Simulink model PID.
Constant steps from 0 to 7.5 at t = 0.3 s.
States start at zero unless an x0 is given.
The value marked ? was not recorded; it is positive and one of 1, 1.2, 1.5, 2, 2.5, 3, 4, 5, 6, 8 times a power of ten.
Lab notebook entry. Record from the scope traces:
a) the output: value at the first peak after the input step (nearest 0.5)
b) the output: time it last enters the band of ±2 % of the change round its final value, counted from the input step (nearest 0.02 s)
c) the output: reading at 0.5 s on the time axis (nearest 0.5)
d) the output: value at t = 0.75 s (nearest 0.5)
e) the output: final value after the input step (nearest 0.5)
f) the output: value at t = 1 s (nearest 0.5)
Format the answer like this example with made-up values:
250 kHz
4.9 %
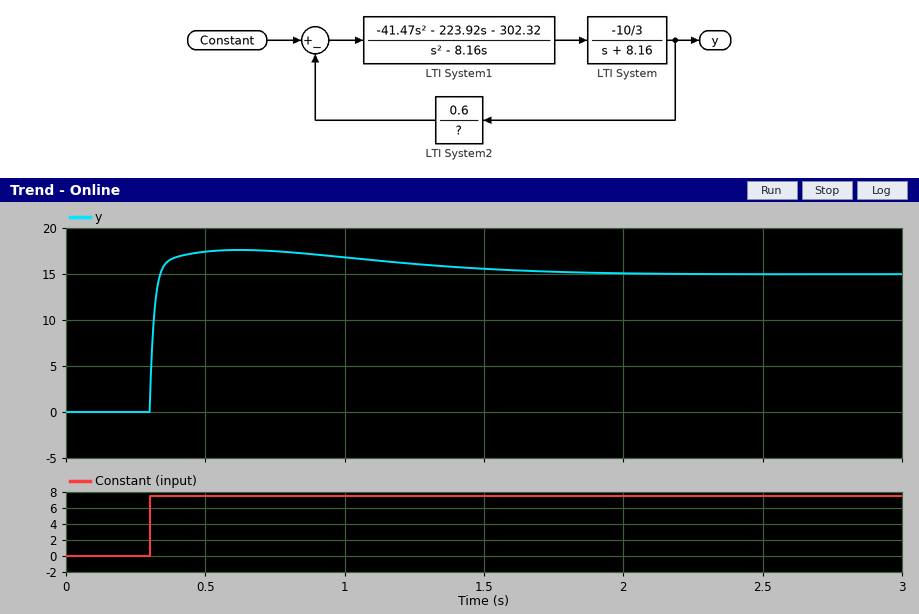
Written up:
17.5
1.40 s
17.5
17.5
15.0
17.0
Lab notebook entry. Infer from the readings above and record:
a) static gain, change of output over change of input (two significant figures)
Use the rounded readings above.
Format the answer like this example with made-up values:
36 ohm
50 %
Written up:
2.0
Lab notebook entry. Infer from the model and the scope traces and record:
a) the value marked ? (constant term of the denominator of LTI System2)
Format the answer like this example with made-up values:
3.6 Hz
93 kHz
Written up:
1.2
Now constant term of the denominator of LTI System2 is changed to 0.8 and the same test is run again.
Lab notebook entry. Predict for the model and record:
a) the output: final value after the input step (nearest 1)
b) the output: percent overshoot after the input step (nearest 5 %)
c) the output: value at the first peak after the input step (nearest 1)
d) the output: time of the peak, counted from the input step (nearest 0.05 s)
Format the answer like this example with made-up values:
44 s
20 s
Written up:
10
10 %
11
0.30 s
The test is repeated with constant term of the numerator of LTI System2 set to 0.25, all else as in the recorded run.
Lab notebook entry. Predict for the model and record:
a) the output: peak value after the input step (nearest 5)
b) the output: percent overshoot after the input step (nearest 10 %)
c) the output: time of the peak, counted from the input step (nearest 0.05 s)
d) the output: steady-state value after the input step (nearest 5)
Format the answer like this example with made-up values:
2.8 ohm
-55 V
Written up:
55
50 %
0.40 s
35
